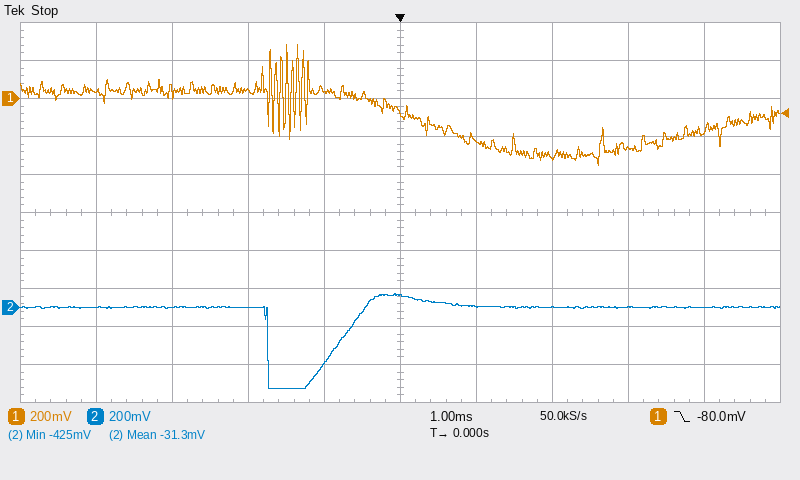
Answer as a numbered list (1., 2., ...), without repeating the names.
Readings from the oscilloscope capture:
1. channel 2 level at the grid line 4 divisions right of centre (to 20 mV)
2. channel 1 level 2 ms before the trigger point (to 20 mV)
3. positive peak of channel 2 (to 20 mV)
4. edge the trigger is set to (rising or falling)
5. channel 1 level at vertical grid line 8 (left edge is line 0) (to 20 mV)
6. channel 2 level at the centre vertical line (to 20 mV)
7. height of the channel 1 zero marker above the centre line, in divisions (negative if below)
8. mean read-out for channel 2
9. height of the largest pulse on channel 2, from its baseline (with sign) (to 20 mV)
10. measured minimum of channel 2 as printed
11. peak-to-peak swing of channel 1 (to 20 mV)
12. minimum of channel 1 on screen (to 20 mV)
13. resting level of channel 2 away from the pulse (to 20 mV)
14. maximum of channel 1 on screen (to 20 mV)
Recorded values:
1. 0 mV
2. 40 mV
3. 80 mV
4. falling
5. -260 mV
6. 60 mV
7. +3.0 div
8. -31.3 mV
9. -420 mV
10. -425 mV
11. 640 mV
12. -360 mV
13. 0 mV
14. 280 mV
